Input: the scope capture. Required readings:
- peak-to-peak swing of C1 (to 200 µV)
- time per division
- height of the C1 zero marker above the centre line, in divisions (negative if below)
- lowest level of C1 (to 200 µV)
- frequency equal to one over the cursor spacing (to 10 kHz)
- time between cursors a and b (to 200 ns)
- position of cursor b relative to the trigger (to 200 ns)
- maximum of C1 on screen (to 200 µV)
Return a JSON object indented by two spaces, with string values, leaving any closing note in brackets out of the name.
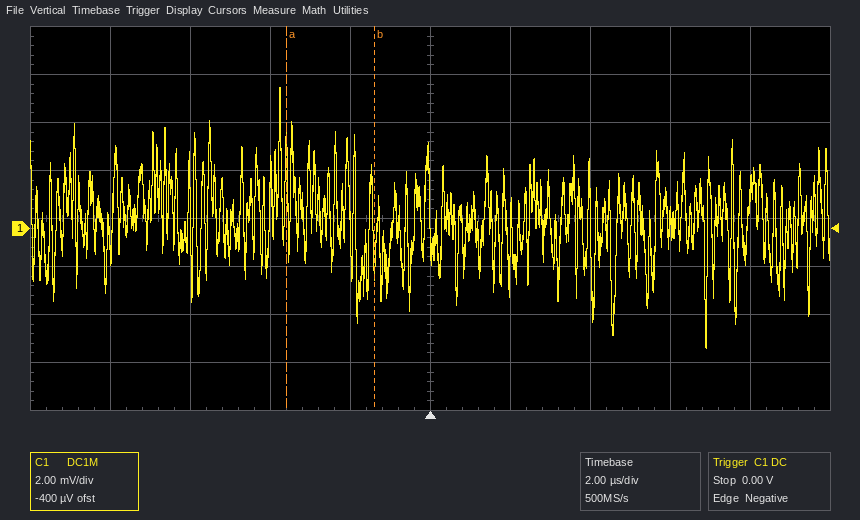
{
  "peak-to-peak swing of C1": "10.8 mV",
  "time per division": "2 µs",
  "height of the C1 zero marker above the centre line, in divisions": "-0.2 div",
  "lowest level of C1": "-5.0 mV",
  "frequency equal to one over the cursor spacing": "450 kHz",
  "time between cursors a and b": "2.2 µs",
  "position of cursor b relative to the trigger": "-1.4 µs",
  "maximum of C1 on screen": "5.8 mV"
}
